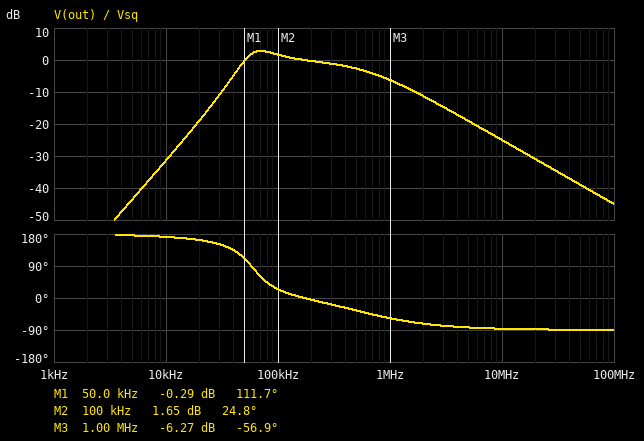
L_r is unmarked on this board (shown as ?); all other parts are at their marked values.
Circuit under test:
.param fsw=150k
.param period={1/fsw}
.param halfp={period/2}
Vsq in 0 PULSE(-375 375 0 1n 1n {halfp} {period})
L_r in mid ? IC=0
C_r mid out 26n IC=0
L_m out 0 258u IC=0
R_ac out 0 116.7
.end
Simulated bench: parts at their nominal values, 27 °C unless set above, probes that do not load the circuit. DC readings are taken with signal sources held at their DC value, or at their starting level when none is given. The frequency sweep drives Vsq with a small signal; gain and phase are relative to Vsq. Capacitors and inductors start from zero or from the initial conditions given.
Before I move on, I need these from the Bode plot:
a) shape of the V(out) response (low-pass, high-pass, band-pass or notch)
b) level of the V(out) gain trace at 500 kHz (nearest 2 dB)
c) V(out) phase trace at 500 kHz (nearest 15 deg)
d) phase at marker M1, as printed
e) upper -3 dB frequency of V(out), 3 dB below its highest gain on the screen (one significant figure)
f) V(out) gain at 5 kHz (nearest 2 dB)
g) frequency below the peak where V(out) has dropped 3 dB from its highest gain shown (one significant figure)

band-pass
-2 dB
-30 deg
111.7 deg
200 kHz
-44 dB
50 kHz
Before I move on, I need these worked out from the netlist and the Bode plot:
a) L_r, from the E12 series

33 µH
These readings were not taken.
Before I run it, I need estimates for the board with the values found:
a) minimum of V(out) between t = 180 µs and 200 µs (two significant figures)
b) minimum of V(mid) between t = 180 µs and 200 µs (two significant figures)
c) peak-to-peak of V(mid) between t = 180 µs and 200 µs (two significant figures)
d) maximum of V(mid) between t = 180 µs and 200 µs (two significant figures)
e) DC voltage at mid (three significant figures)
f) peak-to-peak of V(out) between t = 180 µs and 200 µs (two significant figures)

-480 V
-390 V
780 V
390 V
-375 V
950 V
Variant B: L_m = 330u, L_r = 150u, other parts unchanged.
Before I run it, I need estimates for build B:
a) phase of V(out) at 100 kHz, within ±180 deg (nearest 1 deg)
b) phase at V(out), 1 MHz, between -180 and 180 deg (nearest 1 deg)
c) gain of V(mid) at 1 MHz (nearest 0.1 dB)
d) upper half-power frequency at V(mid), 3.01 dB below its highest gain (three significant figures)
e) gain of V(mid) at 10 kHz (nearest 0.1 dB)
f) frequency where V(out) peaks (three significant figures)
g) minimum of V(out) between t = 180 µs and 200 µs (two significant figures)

-14 deg
-80 deg
-18.2 dB
63.3 kHz
0.1 dB
52.5 kHz
-270 V
